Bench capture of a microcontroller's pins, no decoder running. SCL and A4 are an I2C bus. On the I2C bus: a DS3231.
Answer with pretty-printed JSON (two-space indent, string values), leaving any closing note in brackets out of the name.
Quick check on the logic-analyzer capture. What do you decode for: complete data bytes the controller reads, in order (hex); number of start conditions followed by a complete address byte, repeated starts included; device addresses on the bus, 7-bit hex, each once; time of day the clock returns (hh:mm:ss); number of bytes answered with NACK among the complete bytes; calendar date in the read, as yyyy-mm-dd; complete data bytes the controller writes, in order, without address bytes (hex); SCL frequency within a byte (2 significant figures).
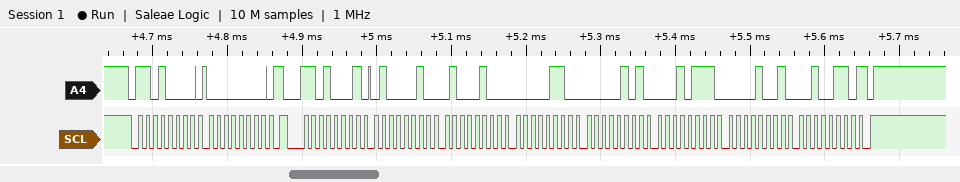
{
  "complete data bytes the controller reads, in order": "42 44 06 05 17 09 26",
  "number of start conditions followed by a complete address byte, repeated starts included": "2",
  "device addresses on the bus, 7-bit hex, each once": "0x68",
  "time of day the clock returns": "06:44:42",
  "number of bytes answered with NACK among the complete bytes": "1",
  "calendar date in the read, as yyyy-mm-dd": "2026-09-17",
  "complete data bytes the controller writes, in order, without address bytes": "00",
  "SCL frequency within a byte": "100 kHz"
}
